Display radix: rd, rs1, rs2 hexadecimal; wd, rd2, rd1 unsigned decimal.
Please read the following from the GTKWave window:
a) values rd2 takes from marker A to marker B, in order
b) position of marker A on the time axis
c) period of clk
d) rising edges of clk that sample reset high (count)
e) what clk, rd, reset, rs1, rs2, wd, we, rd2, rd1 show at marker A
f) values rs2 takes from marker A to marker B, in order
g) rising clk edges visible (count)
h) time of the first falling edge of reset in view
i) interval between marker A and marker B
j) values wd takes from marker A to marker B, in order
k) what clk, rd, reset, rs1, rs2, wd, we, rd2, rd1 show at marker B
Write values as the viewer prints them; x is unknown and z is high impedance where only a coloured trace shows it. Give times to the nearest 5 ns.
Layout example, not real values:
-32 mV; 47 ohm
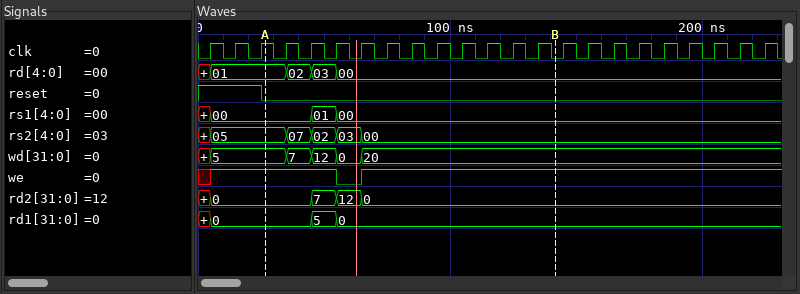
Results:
0, 7, 12, 0; 25 ns; 10 ns; 3; clk=1, rd=01, reset=0, rs1=00, rs2=05, wd=5, we=1, rd2=0, rd1=0; 05, 07, 02, 03, 00; 23; 25 ns; 115 ns; 5, 7, 12, 0, 20; clk=0, rd=00, reset=0, rs1=00, rs2=00, wd=20, we=1, rd2=0, rd1=0
